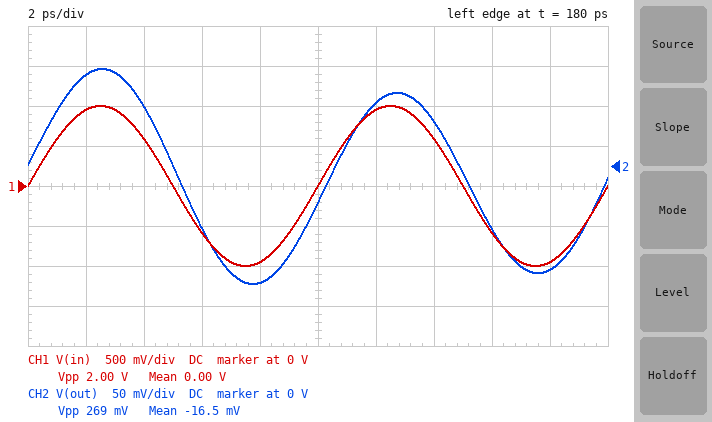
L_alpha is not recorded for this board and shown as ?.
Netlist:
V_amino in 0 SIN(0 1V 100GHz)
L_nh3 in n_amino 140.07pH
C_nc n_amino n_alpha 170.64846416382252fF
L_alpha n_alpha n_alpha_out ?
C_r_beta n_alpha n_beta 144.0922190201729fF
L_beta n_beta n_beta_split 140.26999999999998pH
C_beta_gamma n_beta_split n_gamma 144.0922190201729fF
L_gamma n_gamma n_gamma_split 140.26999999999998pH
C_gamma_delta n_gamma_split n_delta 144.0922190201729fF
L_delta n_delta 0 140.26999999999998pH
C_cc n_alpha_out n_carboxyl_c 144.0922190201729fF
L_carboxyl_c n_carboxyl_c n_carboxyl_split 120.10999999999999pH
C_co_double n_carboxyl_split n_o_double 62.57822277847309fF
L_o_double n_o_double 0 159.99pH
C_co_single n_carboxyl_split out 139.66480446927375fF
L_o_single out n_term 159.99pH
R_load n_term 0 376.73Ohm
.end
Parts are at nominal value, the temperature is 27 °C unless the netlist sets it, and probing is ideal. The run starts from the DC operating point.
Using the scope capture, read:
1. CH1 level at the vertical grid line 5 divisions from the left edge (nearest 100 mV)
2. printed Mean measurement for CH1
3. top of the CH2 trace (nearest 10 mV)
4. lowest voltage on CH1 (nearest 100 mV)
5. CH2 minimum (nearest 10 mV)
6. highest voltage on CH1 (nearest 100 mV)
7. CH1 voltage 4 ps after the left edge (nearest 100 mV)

0 V
0.00 V
120 mV
-1.0 V
-150 mV
1.0 V
600 mV
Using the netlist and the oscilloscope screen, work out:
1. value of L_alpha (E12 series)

390 pH
